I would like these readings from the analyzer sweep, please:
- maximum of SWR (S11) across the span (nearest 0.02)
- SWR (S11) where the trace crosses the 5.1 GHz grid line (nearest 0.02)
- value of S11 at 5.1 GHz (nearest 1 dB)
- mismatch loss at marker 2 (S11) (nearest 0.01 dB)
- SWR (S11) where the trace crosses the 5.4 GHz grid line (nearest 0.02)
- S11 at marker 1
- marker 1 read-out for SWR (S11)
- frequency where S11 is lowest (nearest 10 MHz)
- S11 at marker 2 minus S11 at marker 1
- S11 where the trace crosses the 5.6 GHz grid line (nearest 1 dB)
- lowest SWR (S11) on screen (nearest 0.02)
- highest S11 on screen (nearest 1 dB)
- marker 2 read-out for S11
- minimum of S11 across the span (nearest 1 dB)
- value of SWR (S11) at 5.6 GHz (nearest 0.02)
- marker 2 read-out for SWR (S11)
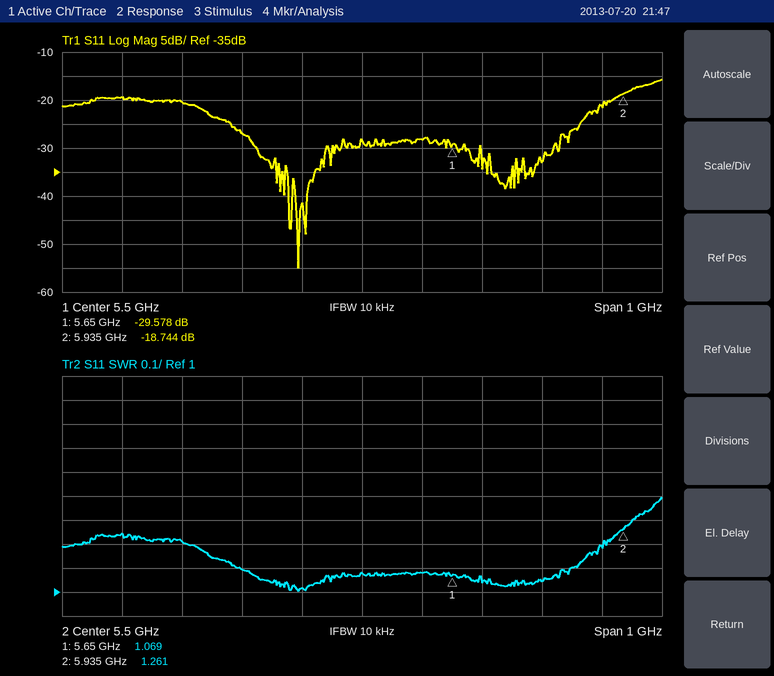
1.40
1.24
-19 dB
0.06 dB
1.02
-29.578 dB
1.069
5.39 GHz
10.834 dB
-28 dB
1.00
-16 dB
-18.744 dB
-55 dB
1.08
1.261
